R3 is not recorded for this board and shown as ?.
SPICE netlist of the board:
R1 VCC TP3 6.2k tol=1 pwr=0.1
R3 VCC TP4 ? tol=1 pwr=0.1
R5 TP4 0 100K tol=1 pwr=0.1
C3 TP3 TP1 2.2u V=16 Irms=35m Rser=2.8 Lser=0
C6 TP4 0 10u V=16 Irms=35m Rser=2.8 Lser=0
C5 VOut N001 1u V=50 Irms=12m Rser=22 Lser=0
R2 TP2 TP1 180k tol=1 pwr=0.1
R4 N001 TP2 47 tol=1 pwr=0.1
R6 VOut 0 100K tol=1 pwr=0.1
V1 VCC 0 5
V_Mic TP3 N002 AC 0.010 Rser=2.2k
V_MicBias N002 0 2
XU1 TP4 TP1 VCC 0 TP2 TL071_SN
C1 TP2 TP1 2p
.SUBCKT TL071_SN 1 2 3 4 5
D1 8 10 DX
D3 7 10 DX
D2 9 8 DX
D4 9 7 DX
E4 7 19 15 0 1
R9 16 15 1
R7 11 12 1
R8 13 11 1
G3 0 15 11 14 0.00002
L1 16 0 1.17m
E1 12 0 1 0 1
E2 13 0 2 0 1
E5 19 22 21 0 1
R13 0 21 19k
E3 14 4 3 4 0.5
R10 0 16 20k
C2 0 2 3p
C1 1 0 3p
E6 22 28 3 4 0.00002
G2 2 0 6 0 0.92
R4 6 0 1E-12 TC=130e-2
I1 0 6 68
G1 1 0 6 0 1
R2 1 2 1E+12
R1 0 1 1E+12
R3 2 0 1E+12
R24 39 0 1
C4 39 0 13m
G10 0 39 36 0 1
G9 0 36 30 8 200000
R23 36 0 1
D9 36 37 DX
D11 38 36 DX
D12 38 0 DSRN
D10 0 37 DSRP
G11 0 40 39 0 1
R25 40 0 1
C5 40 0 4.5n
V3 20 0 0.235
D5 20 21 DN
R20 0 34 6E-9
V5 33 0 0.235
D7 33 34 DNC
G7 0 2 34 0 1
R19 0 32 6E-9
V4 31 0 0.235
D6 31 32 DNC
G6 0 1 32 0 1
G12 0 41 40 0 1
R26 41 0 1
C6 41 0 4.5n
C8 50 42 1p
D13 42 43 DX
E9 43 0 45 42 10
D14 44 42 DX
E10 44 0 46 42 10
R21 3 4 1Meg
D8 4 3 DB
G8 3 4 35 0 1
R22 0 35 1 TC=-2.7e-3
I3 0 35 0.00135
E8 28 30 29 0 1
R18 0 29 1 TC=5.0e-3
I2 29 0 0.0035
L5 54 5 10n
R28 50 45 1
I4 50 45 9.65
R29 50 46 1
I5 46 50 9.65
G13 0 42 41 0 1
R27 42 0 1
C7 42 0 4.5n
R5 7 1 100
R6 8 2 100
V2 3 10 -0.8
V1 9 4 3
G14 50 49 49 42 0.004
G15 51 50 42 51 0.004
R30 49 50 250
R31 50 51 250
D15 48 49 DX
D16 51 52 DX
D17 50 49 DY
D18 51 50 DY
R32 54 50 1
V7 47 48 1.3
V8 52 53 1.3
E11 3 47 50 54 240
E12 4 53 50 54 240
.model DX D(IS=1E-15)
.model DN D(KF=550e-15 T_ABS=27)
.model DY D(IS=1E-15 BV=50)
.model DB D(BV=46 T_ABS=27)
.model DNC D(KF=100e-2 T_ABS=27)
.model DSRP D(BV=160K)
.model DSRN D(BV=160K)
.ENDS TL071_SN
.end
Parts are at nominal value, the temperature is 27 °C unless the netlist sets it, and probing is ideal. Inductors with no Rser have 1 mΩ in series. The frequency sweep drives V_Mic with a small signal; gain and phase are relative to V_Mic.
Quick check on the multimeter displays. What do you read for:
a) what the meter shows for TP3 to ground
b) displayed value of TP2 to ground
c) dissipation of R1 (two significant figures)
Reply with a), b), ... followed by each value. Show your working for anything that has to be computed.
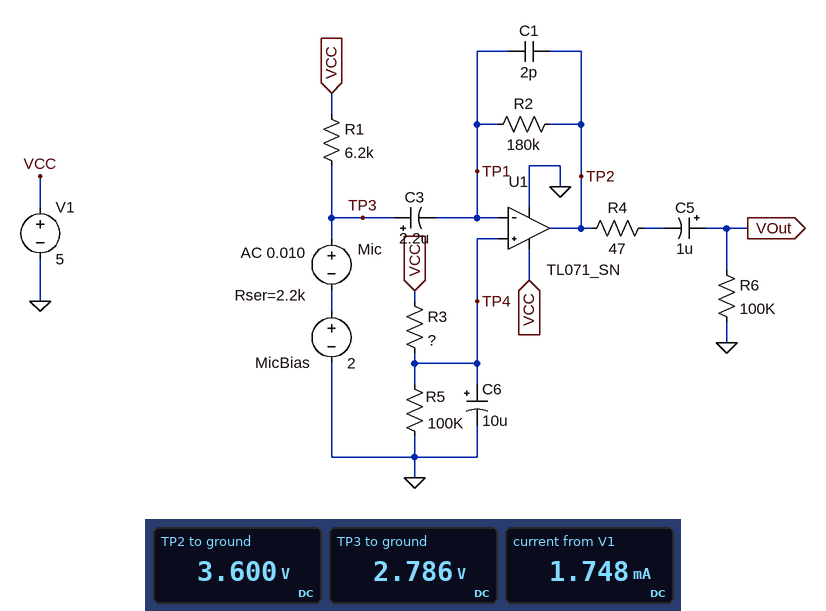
a) 2.786 V
b) 3.600 V
c) (5 V - 2.786 V)^2 / 6.2 kΩ = 790 µW
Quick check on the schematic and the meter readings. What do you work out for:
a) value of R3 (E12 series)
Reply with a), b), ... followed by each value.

a) 39 kΩ
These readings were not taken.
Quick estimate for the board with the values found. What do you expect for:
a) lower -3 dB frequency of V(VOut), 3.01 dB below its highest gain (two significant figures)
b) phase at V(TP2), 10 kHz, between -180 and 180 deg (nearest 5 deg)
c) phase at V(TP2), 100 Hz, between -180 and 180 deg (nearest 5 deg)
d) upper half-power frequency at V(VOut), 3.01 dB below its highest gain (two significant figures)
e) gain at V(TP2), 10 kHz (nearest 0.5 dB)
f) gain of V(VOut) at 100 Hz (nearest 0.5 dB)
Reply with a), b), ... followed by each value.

a) 44 Hz
b) 155 deg
c) -155 deg
d) 21 kHz
e) 37.5 dB
f) 37.5 dB
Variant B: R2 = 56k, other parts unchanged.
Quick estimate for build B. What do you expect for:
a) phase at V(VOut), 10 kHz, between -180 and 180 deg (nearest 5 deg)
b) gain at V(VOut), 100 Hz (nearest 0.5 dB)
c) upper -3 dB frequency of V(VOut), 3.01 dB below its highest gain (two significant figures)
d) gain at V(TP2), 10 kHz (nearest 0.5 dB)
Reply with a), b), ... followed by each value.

a) 170 deg
b) 27.5 dB
c) 66 kHz
d) 28.0 dB
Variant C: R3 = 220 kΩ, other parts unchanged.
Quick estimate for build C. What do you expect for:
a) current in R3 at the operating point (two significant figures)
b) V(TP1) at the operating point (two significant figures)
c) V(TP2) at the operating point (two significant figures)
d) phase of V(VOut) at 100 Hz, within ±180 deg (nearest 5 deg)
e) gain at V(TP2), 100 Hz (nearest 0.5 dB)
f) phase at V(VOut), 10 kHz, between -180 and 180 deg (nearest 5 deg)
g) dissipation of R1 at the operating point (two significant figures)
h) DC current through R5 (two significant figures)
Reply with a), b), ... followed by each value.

a) 12 µA
b) 2.4 V
c) 1.1 V
d) 10 deg
e) -40.0 dB
f) 0 deg
g) 790 µW
h) 24 µA
